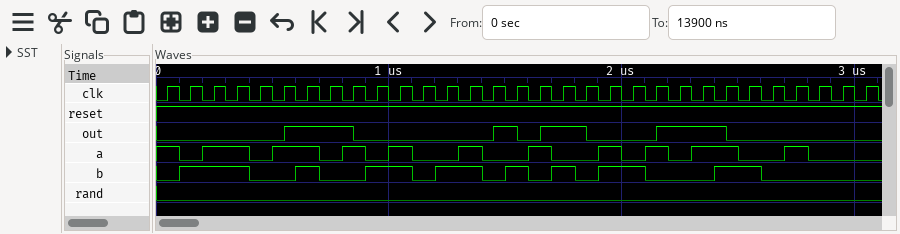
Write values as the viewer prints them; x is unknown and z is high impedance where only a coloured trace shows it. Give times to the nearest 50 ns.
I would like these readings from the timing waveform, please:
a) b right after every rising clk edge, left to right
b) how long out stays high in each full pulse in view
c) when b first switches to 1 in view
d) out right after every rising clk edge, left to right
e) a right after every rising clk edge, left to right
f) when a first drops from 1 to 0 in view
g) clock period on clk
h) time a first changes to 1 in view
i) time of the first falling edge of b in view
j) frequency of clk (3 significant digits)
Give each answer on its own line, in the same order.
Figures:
0 1 1 1 0 0 1 0 0 1 1 0 1 1 0 1 0 1 0 1 1 0 0 0 1 1 0 0 0 0 0
300 ns, 100 ns, 200 ns, 300 ns
100 ns
0 0 0 0 0 1 1 1 0 0 0 0 0 0 1 0 1 1 0 0 0 1 1 1 0 0 0 0 0 0 0
1 0 1 1 0 1 1 0 1 0 1 0 0 1 0 0 1 0 0 1 0 1 0 1 1 0 0 1 0 0 0
100 ns
100 ns
200 ns
400 ns
10.0 MHz
